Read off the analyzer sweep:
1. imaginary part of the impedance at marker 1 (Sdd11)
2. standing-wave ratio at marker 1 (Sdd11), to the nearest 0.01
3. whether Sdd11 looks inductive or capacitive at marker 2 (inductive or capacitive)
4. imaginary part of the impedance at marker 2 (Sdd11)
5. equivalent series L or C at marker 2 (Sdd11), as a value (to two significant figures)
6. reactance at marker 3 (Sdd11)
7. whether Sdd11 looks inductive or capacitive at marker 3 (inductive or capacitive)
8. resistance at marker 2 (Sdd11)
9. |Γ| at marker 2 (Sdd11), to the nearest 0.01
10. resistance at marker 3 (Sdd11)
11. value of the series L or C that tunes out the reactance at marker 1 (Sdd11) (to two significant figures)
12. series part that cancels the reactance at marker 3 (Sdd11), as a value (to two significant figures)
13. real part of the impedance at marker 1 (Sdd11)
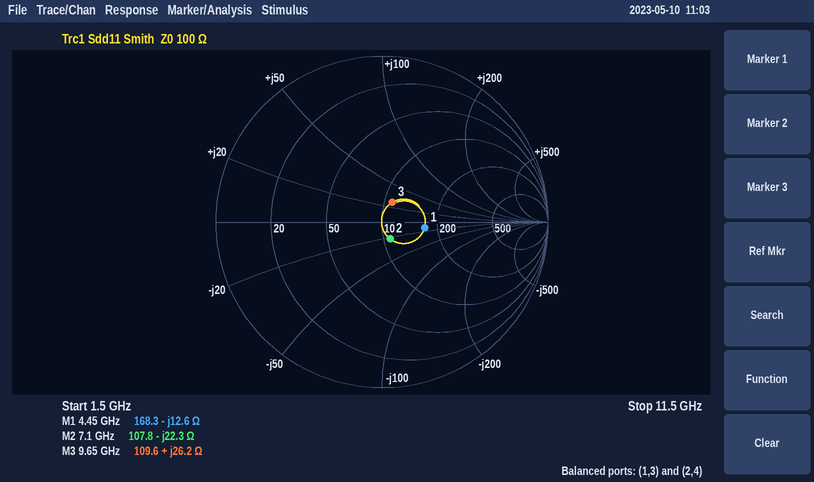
-12.6 Ω
1.70
capacitive
-22.3 Ω
1.0 pF
+26.2 Ω
inductive
107.8 Ω
0.11
109.6 Ω
450 pH
630 fF
168.3 Ω
